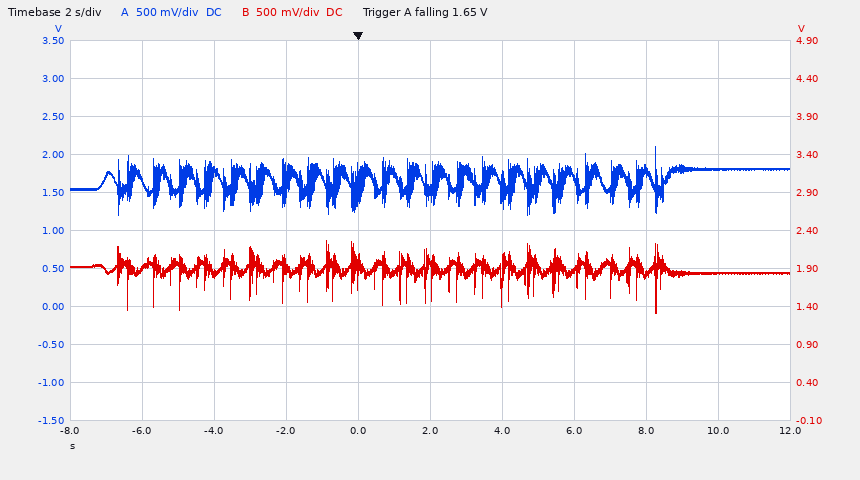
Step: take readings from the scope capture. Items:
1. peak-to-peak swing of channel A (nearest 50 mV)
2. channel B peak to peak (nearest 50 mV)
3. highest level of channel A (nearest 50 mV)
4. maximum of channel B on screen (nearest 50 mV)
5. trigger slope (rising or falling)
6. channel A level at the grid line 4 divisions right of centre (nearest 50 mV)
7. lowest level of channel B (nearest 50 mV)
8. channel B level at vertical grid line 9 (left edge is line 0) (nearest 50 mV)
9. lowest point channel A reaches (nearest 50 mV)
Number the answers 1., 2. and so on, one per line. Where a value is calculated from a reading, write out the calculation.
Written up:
1. 2.10 V − (1.20 V) = 900 mV
2. 2.25 V − (1.30 V) = 950 mV
3. 2.10 V
4. 2.25 V
5. falling
6. 1.80 V
7. 1.30 V
8. 1.85 V
9. 1.20 V
